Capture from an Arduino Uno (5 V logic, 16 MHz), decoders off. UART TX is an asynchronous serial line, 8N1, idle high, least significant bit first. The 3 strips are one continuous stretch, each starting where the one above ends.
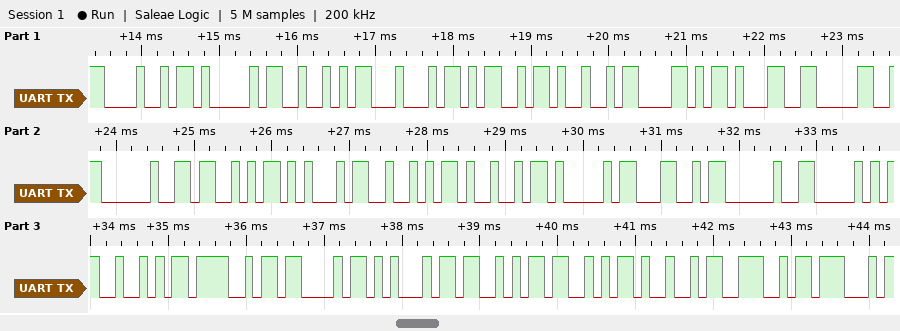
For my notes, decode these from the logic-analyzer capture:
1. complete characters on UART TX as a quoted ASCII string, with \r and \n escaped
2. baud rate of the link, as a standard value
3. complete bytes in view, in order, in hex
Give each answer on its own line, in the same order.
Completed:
"HARDMIX10 SERIAL PROCESSING"
9600 baud
48 41 52 44 4D 49 58 31 30 20 53 45 52 49 41 4C 20 50 52 4F 43 45 53 53 49 4E 47
